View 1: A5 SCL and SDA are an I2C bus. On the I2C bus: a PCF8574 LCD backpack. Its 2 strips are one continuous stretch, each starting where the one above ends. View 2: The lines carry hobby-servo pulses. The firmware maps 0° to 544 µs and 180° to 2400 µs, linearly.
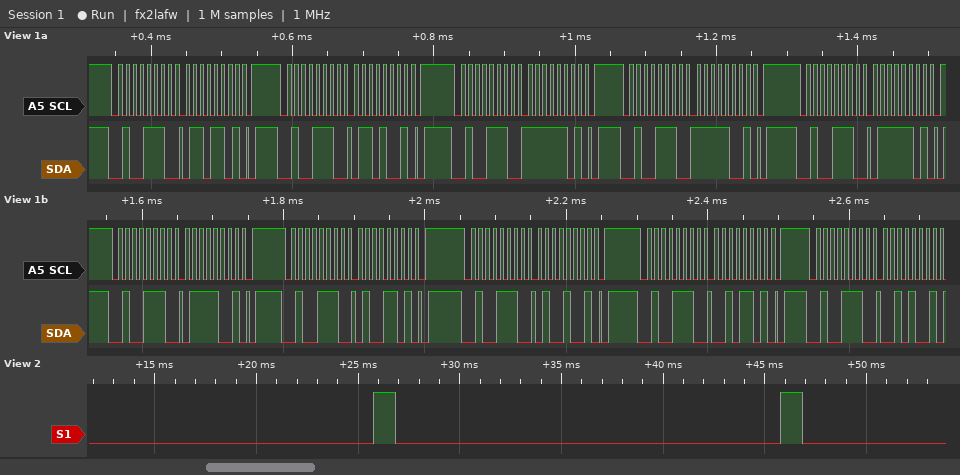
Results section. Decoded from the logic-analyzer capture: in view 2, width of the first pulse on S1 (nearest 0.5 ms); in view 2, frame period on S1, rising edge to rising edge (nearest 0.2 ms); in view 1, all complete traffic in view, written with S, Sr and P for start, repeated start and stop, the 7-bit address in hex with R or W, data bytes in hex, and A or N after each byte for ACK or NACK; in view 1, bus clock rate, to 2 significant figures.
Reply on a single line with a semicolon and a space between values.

1.0 ms; 20.0 ms; S 27W A 6D A P S 27W A 69 A P S 27W A FD A P S 27W A F9 A P S 27W A 7D A P S 27W A 79 A P S 27W A 4D A P S 27W A 49 A P S 27W A 2D A P S 27W A 29 A; 100 kHz
